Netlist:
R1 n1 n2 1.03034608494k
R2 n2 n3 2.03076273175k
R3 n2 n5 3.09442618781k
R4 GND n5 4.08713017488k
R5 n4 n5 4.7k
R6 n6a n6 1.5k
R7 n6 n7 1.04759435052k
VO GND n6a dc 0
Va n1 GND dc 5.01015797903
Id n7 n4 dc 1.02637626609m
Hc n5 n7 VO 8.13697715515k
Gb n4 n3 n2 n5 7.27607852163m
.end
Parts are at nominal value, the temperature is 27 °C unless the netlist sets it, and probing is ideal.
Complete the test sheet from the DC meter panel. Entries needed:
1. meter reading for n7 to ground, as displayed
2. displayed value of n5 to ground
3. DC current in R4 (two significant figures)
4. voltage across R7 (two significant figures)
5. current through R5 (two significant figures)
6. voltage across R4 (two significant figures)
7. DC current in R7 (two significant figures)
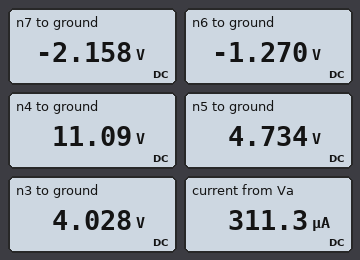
-2.158 V
4.734 V
1.2 mA
890 mV
1.4 mA
4.7 V
850 µA
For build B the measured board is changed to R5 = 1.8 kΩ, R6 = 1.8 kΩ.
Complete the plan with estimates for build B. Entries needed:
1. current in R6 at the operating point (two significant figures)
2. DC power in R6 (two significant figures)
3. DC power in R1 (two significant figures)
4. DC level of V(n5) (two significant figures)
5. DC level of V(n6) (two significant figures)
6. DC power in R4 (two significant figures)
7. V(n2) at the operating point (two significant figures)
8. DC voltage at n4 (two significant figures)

900 µA
1.5 mW
73 µW
4.8 V
-1.6 V
5.6 mW
4.7 V
7.1 V
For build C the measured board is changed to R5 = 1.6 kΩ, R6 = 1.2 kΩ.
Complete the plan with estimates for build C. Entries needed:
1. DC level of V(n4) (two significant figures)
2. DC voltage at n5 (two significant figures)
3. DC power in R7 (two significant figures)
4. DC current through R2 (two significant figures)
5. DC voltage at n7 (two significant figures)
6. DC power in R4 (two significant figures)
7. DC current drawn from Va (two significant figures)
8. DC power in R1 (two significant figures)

6.9 V
4.7 V
670 µW
370 µA
-1.8 V
5.4 mW
350 µA
130 µW
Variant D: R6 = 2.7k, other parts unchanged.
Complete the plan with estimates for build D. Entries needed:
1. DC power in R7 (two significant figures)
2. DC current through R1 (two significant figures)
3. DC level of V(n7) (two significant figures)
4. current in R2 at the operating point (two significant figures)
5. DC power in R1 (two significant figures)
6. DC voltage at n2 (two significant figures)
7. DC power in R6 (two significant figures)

1.3 mW
83 µA
-4.2 V
87 µA
7.1 µW
4.9 V
3.4 mW
